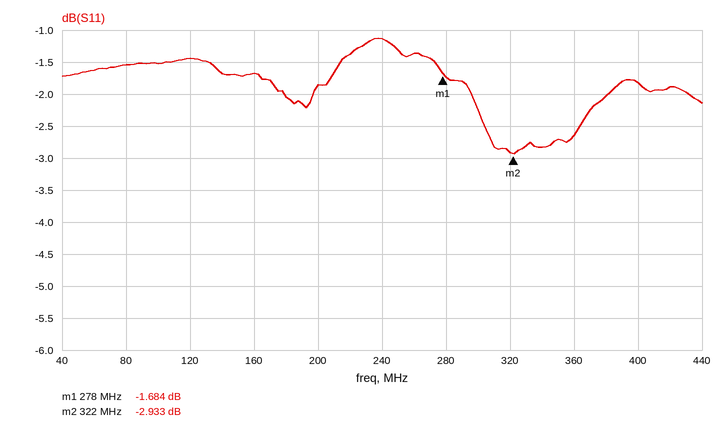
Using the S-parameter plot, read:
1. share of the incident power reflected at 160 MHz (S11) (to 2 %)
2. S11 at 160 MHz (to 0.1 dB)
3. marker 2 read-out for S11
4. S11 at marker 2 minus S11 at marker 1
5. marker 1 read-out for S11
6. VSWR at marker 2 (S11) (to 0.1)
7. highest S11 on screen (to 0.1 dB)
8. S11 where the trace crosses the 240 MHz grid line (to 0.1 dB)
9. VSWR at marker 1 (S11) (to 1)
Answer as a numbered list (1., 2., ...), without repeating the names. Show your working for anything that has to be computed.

1. 10^(-1.7/10) ≈ 68 %
2. -1.7 dB
3. -2.933 dB
4. -2.933 − (-1.684) = -1.249 dB
5. -1.684 dB
6. (1 + 0.7134)/(1 − 0.7134) ≈ 6.0
7. -1.1 dB
8. -1.1 dB
9. (1 + 0.8238)/(1 − 0.8238) ≈ 10
